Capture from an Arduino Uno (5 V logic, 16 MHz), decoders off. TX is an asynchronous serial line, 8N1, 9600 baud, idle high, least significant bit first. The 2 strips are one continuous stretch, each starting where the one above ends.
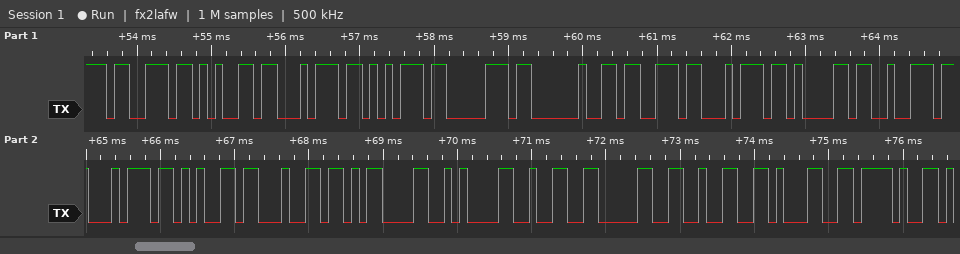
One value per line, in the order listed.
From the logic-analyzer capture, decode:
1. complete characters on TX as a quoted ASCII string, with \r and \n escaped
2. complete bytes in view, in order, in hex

"setup started\r\n2021/"
73 65 74 75 70 20 73 74 61 72 74 65 64 0D 0A 32 30 32 31 2F
